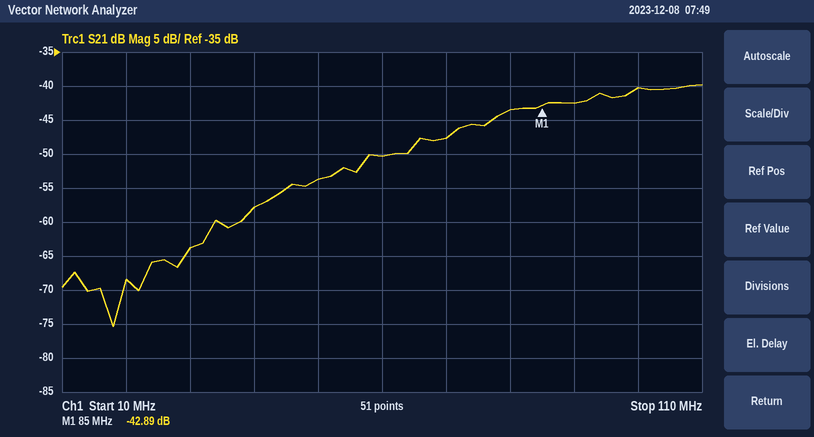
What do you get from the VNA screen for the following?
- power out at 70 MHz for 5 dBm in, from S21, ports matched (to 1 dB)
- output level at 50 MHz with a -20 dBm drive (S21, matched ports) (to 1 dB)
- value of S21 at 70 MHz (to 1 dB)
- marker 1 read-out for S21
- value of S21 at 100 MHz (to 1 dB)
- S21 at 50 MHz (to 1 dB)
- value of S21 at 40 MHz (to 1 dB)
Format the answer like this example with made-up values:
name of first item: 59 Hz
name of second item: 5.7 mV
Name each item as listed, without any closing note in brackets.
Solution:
power out at 70 MHz for 5 dBm in, from S21, ports matched: -43 dBm
output level at 50 MHz with a -20 dBm drive (S21, matched ports): -74 dBm
value of S21 at 70 MHz: -48 dB
marker 1 read-out for S21: -42.89 dB
value of S21 at 100 MHz: -40 dB
S21 at 50 MHz: -54 dB
value of S21 at 40 MHz: -58 dB
